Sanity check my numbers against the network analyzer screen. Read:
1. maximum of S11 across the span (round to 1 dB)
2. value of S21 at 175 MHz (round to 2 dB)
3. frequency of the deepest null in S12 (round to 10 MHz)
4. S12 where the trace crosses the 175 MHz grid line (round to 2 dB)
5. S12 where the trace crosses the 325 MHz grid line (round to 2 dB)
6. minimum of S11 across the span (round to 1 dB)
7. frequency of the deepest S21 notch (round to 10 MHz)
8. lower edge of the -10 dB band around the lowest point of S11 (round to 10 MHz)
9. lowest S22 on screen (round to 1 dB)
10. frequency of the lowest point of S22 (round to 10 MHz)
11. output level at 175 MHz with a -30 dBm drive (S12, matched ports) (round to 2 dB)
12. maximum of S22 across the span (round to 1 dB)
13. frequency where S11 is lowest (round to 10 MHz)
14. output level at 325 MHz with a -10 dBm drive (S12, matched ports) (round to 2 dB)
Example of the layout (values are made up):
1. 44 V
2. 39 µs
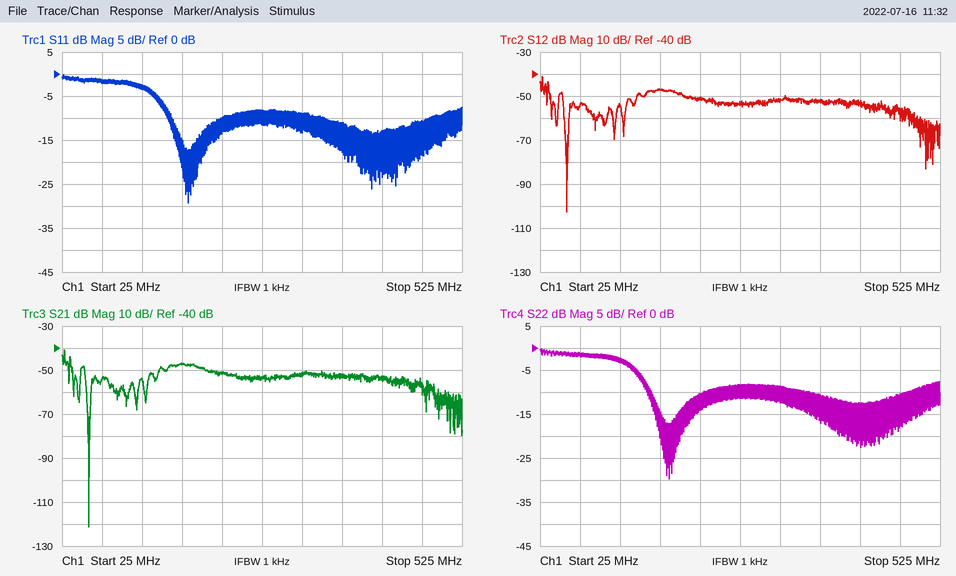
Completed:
1. 0 dB
2. -48 dB
3. 60 MHz
4. -48 dB
5. -52 dB
6. -29 dB
7. 60 MHz
8. 160 MHz
9. -30 dB
10. 190 MHz
11. -78 dBm
12. 0 dB
13. 180 MHz
14. -62 dBm
